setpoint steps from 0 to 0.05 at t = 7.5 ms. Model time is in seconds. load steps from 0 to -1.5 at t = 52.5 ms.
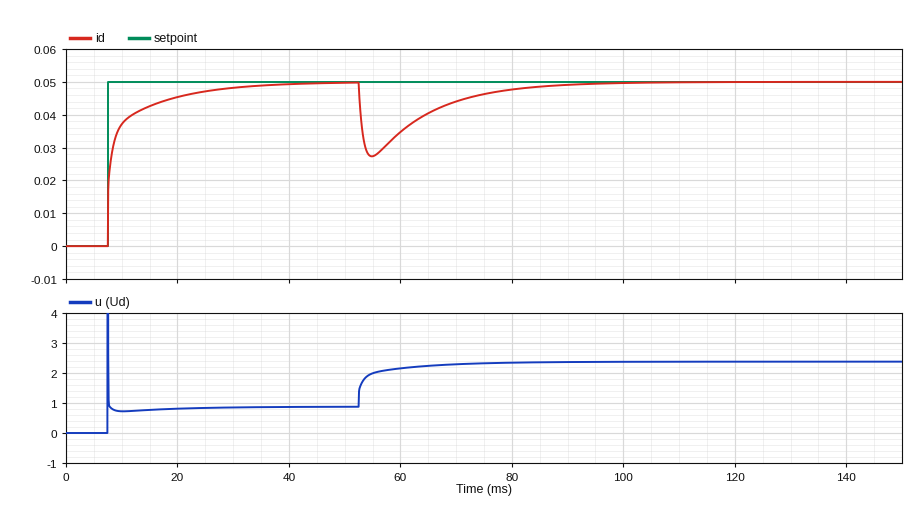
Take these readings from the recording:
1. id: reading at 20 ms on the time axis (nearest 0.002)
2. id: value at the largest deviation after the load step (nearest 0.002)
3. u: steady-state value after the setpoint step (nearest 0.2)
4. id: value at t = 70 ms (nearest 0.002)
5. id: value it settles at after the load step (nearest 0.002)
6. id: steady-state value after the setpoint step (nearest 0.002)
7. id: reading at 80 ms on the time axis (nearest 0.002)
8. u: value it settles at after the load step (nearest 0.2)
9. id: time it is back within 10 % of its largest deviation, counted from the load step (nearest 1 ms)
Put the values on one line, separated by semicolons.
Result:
0.046; 0.028; 0.8; 0.044; 0.050; 0.050; 0.048; 2.4; 28 ms
